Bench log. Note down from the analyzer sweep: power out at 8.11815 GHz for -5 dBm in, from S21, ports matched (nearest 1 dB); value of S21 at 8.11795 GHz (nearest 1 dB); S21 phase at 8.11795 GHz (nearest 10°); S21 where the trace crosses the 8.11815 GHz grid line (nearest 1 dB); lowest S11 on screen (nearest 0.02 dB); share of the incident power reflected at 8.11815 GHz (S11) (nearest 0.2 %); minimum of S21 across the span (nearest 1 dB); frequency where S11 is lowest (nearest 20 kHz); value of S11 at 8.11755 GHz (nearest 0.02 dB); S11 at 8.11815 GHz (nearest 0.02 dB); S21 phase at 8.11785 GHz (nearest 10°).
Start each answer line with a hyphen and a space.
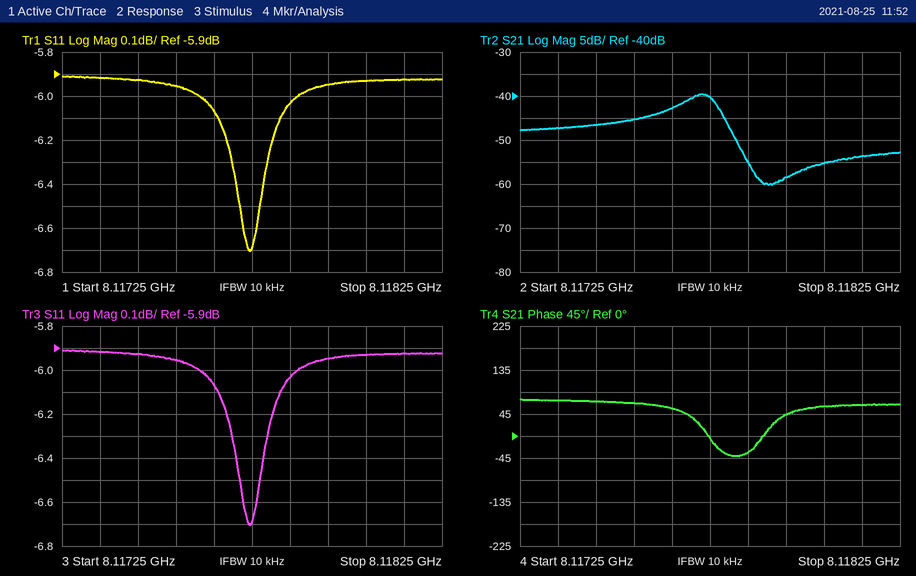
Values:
- -59 dBm
- -58 dB
- 40°
- -54 dB
- -6.70 dB
- 25.6 %
- -60 dB
- 8.11774 GHz
- -5.96 dB
- -5.92 dB
- -30°
